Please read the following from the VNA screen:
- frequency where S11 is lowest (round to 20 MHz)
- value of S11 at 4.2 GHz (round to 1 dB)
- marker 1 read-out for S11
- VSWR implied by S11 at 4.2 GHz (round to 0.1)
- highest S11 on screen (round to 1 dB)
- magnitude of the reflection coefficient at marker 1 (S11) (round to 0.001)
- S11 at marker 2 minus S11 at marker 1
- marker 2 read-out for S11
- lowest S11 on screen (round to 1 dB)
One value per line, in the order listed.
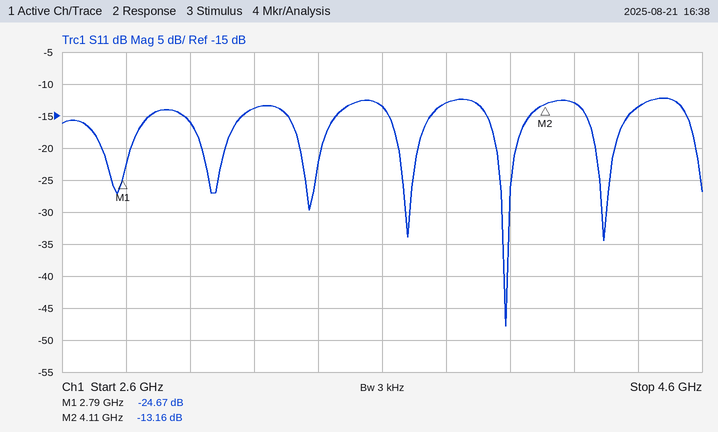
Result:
3.98 GHz
-13 dB
-24.67 dB
1.6
-12 dB
0.058
11.51 dB
-13.16 dB
-48 dB
